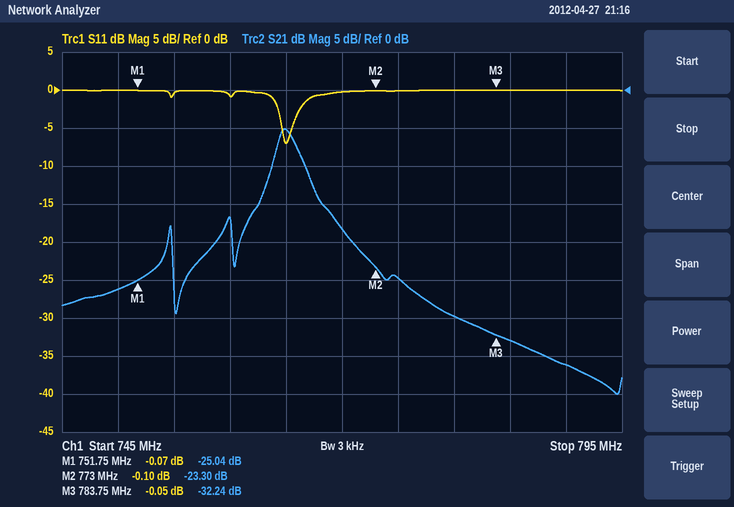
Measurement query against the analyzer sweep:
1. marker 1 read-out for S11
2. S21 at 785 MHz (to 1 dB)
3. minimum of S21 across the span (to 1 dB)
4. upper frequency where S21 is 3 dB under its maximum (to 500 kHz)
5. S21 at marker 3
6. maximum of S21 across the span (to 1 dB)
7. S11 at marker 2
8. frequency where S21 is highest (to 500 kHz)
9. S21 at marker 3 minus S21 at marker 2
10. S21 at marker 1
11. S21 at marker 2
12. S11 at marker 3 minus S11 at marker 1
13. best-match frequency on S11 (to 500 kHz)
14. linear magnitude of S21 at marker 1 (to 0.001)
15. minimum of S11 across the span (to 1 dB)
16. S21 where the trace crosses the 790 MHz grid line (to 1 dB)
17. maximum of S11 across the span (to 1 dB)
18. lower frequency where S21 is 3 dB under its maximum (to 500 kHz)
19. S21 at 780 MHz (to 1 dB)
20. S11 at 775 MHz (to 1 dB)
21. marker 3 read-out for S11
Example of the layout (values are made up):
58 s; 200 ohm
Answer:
-0.07 dB; -33 dB; -40 dB; 766.0 MHz; -32.24 dB; -5 dB; -0.10 dB; 765.0 MHz; -8.94 dB; -25.04 dB; -23.30 dB; 0.02 dB; 765.0 MHz; 0.056; -7 dB; -36 dB; 0 dB; 764.0 MHz; -30 dB; 0 dB; -0.05 dB
